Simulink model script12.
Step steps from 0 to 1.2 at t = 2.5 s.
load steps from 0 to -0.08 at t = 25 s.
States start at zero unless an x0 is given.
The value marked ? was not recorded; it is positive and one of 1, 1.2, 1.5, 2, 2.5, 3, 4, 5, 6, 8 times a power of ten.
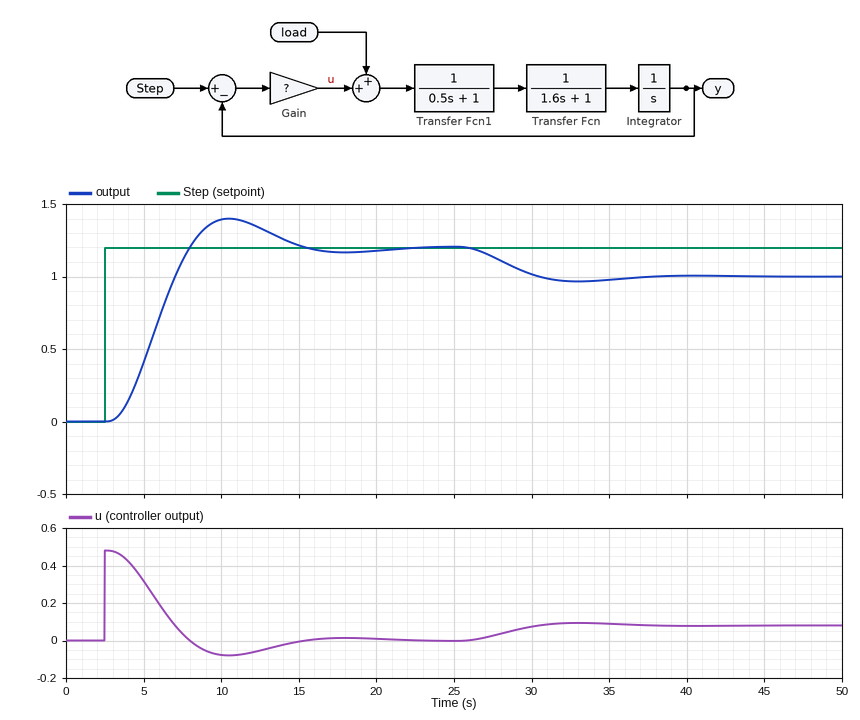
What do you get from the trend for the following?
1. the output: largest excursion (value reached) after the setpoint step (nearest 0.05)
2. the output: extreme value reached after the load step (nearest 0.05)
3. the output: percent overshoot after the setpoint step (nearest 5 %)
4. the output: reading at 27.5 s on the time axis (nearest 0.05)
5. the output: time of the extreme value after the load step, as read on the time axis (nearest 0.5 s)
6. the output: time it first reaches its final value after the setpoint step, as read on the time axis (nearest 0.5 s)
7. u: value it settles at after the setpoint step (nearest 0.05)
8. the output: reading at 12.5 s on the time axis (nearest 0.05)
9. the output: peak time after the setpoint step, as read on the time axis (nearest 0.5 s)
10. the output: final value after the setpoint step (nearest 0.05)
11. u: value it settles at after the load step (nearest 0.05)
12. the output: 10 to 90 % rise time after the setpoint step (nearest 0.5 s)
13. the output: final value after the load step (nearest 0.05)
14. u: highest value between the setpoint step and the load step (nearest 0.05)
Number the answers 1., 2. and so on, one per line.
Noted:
1. 1.40
2. 0.95
3. 15 %
4. 1.15
5. 33.0 s
6. 8.0 s
7. 0.00
8. 1.35
9. 10.5 s
10. 1.20
11. 0.10
12. 3.5 s
13. 1.00
14. 0.50
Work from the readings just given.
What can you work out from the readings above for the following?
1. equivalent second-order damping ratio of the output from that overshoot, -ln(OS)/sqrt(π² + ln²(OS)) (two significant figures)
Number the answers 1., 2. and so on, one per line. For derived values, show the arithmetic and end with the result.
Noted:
1. ln(0.15) = -1.897; 1.897 / sqrt(9.870 + 3.599) = 0.52
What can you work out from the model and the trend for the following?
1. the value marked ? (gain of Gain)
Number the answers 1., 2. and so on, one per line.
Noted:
1. 0.4
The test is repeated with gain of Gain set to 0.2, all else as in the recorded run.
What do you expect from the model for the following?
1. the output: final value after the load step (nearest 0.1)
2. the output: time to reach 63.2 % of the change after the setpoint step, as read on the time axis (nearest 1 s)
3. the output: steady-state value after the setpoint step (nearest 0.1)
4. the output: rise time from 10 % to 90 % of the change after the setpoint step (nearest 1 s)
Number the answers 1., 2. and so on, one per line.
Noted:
1. 0.8
2. 8 s
3. 1.2
4. 7 s
